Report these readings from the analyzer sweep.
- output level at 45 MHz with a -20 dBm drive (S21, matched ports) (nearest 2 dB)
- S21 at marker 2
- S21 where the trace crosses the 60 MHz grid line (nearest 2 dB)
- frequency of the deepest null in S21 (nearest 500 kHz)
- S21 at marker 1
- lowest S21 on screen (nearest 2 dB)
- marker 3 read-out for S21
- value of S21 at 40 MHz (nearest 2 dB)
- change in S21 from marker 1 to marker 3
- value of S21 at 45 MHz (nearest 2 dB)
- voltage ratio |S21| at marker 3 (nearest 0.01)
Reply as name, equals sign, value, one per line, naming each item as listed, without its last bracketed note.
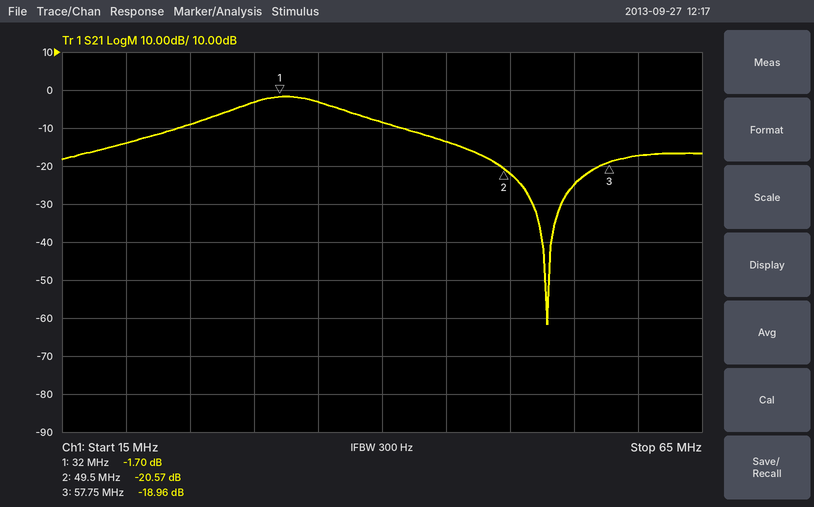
output level at 45 MHz with a -20 dBm drive (S21, matched ports) = -34 dBm
S21 at marker 2 = -20.57 dB
S21 where the trace crosses the 60 MHz grid line = -18 dB
frequency of the deepest null in S21 = 53.0 MHz
S21 at marker 1 = -1.70 dB
lowest S21 on screen = -62 dB
marker 3 read-out for S21 = -18.96 dB
value of S21 at 40 MHz = -8 dB
change in S21 from marker 1 to marker 3 = -17.26 dB
value of S21 at 45 MHz = -14 dB
voltage ratio |S21| at marker 3 = 0.11
